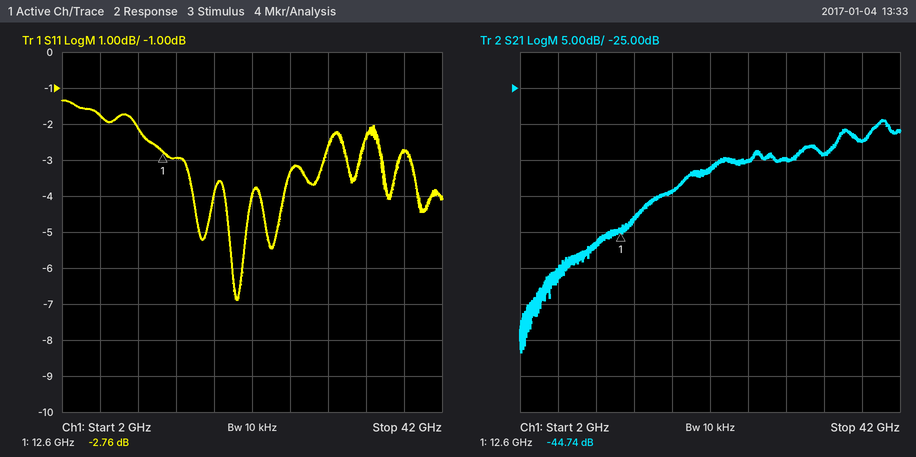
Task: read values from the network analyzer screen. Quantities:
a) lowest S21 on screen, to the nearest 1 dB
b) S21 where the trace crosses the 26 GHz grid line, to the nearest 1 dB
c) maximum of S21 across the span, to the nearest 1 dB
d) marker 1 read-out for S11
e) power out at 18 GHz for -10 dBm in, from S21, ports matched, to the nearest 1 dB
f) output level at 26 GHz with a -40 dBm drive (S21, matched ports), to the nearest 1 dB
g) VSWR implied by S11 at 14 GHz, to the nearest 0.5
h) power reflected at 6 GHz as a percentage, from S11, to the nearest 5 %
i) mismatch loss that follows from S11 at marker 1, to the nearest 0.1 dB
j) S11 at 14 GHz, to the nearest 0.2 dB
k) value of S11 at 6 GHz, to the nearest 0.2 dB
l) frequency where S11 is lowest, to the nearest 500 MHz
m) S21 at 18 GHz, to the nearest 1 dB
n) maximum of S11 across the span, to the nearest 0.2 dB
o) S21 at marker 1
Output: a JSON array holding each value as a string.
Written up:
["-62 dB", "-35 dB", "-29 dB", "-2.76 dB", "-49 dBm", "-75 dBm", "6.0", "65 %", "3.3 dB", "-3.0 dB", "-1.8 dB", "20.5 GHz", "-39 dB", "-1.4 dB", "-44.74 dB"]
